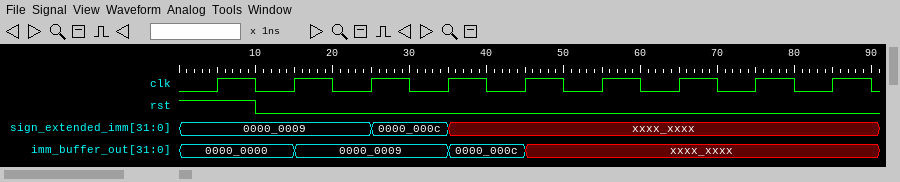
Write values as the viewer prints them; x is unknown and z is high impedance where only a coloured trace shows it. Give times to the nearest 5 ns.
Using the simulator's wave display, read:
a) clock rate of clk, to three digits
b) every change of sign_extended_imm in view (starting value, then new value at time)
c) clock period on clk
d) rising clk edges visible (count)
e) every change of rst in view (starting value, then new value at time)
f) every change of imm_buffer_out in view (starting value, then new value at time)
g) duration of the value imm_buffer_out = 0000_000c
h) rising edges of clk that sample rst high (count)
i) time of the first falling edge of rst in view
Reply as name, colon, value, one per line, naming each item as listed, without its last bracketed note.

clock rate of clk, to three digits: 100 MHz
every change of sign_extended_imm in view: 0000_0009, 0000_000c at 25 ns, xxxx_xxxx at 35 ns
clock period on clk: 10 ns
rising clk edges visible: 9
every change of rst in view: 1, 0 at 10 ns
every change of imm_buffer_out in view: 0000_0000, 0000_0009 at 15 ns, 0000_000c at 35 ns, xxxx_xxxx at 45 ns
duration of the value imm_buffer_out = 0000_000c: 10 ns
rising edges of clk that sample rst high: 1
time of the first falling edge of rst in view: 10 ns
